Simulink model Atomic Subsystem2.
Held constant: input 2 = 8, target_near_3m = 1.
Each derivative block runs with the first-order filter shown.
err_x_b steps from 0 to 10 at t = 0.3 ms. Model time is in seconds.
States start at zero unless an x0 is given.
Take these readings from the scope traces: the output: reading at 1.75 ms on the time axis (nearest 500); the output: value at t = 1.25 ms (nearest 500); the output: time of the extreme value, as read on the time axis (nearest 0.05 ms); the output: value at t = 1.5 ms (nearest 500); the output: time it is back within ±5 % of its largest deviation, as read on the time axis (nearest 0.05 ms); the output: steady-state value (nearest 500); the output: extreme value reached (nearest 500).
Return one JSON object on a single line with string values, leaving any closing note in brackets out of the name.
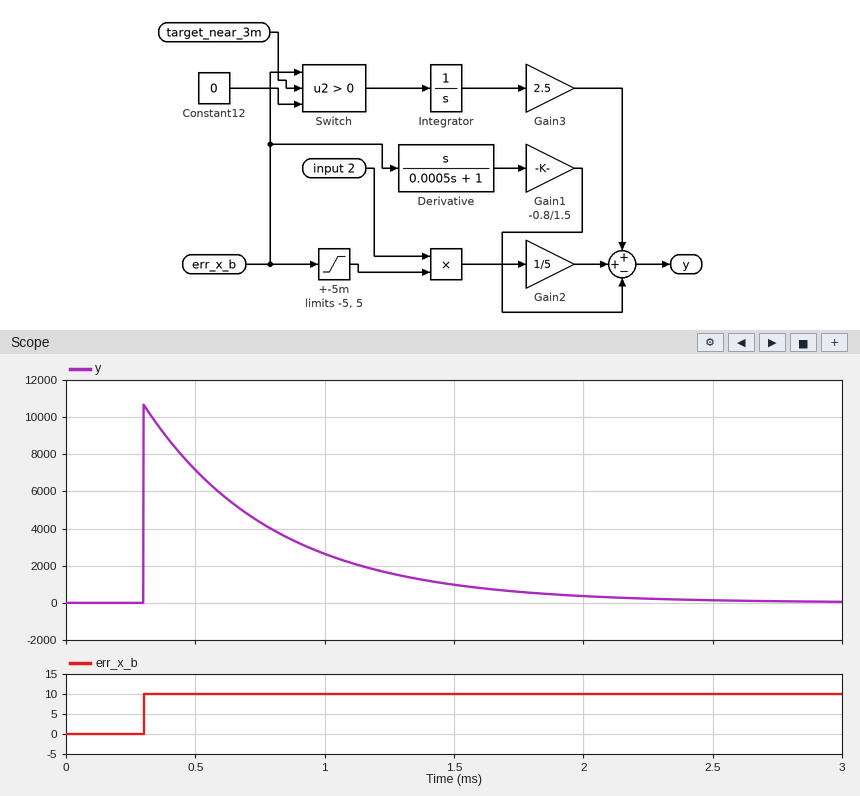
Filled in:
{"the output: reading at 1.75 ms on the time axis": "500", "the output: value at t = 1.25 ms": "1500", "the output: time of the extreme value, as read on the time axis": "0.30 ms", "the output: value at t = 1.5 ms": "1000", "the output: time it is back within ±5 % of its largest deviation, as read on the time axis": "1.80 ms", "the output: steady-state value": "0", "the output: extreme value reached": "10500"}
